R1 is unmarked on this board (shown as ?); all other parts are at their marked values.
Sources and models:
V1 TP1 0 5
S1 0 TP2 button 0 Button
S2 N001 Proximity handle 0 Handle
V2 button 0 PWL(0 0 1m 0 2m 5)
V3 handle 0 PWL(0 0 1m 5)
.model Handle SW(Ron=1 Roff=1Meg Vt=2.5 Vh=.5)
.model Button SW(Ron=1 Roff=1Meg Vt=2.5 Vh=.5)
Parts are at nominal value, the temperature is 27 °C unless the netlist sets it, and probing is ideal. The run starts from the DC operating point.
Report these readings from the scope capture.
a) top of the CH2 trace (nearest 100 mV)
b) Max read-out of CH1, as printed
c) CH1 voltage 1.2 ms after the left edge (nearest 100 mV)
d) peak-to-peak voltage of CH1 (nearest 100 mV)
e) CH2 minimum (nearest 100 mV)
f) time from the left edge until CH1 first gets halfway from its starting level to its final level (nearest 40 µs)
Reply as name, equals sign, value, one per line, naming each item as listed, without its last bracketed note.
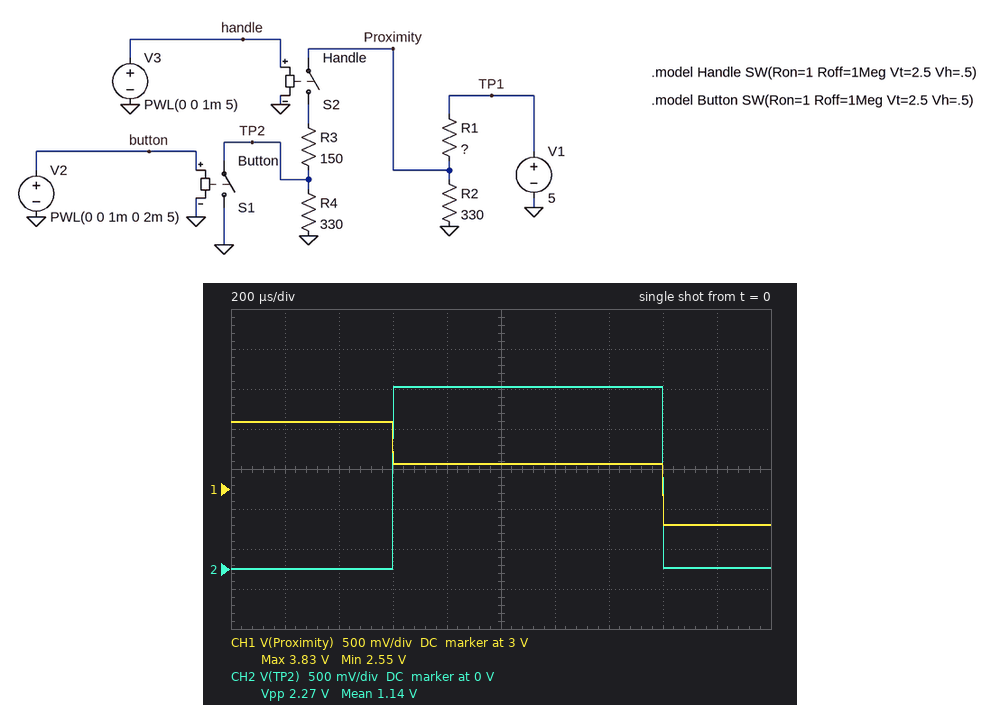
top of the CH2 trace = 2.3 V
Max read-out of CH1, as printed = 3.83 V
CH1 voltage 1.2 ms after the left edge = 3.3 V
peak-to-peak voltage of CH1 = 1.3 V
CH2 minimum = 0 V
time from the left edge until CH1 first gets halfway from its starting level to its final level = 1.60 ms
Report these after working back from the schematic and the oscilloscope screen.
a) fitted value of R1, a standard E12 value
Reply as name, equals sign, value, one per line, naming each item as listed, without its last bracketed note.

fitted value of R1, a standard E12 value = 100 Ω
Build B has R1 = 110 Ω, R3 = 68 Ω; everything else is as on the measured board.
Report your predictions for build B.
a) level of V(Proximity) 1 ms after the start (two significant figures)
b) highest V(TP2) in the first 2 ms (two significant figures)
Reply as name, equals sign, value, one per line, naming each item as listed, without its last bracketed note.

level of V(Proximity) 1 ms after the start = 3.1 V
highest V(TP2) in the first 2 ms = 2.6 V
